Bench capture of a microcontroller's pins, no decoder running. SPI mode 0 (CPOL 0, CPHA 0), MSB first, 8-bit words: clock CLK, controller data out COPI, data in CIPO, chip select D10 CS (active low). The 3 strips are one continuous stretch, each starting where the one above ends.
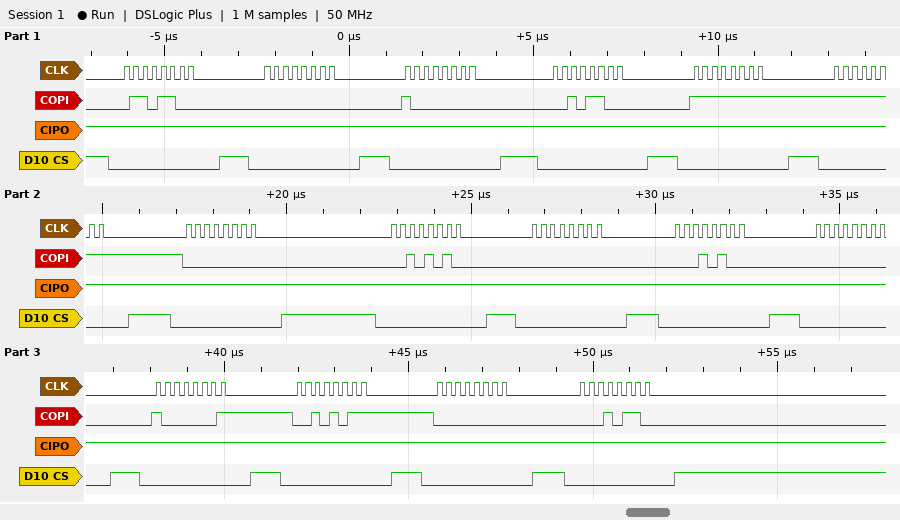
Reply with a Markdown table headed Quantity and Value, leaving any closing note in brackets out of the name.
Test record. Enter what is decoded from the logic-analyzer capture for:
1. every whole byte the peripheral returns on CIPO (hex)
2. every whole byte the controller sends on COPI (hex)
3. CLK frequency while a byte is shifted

| Quantity | Value |
|---|---|
| every whole byte the peripheral returns on CIPO | FF FF FF FF FF FF FF FF FF FF FF FF FF FF FF |
| every whole byte the controller sends on COPI | 6C 00 80 2C FF FF 00 2A 00 14 00 81 2B 00 16 |
| CLK frequency while a byte is shifted | 4 MHz |
